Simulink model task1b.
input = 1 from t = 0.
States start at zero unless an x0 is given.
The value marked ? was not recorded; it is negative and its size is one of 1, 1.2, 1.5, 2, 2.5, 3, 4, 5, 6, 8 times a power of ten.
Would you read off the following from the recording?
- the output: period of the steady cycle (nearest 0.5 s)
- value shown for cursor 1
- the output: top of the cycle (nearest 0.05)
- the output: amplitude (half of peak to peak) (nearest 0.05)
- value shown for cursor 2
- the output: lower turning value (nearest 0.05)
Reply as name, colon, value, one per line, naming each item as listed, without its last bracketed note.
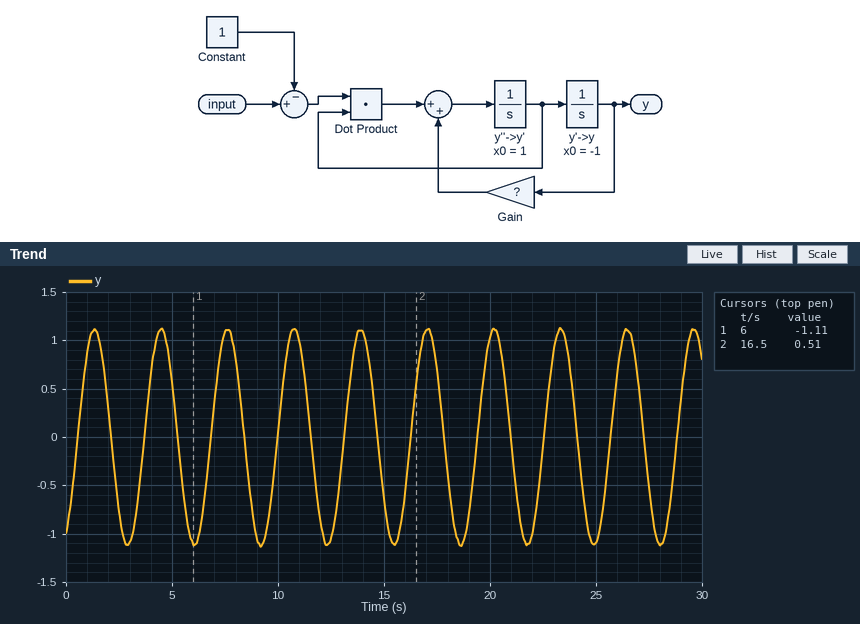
the output: period of the steady cycle: 3.0 s
value shown for cursor 1: -1.11
the output: top of the cycle: 1.10
the output: amplitude (half of peak to peak): 1.10
value shown for cursor 2: 0.51
the output: lower turning value: -1.10
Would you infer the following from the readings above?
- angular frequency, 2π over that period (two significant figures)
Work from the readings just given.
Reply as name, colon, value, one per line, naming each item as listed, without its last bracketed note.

angular frequency, 2π over that period: 2.1 rad/s
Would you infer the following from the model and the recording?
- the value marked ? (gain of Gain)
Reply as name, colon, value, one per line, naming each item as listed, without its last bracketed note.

the value marked ?: -4
